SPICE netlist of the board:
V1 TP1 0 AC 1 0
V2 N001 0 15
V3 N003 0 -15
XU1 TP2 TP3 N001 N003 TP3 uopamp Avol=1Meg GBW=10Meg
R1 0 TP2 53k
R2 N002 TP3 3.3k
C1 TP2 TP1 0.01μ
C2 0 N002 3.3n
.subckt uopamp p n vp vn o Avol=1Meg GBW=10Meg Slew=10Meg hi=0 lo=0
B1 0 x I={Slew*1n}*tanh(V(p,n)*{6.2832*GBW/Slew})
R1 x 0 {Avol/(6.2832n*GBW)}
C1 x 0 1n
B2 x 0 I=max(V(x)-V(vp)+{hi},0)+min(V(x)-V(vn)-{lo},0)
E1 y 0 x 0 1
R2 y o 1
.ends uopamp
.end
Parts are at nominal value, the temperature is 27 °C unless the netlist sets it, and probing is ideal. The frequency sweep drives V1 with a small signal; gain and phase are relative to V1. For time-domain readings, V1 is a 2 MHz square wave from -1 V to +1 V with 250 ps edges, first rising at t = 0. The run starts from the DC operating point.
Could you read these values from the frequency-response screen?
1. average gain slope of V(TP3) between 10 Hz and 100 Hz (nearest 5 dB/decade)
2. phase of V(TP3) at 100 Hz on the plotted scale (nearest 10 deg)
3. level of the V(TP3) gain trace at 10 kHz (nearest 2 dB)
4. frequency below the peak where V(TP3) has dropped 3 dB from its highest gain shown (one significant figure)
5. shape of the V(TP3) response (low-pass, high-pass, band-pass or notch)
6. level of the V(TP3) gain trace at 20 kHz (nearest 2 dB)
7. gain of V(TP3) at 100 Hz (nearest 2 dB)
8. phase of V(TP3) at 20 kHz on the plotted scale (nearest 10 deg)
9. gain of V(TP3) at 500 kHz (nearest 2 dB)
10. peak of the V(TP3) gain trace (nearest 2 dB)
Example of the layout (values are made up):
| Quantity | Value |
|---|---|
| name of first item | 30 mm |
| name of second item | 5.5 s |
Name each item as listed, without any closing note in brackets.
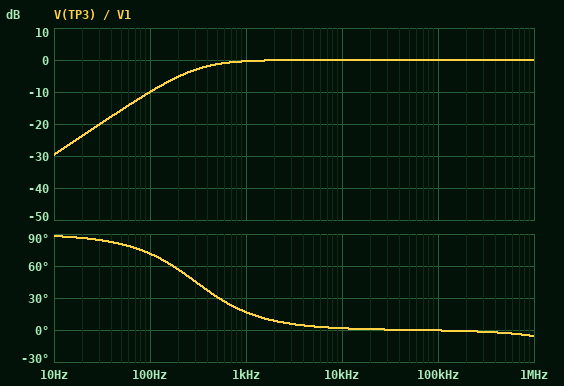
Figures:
| Quantity | Value |
|---|---|
| average gain slope of V(TP3) between 10 Hz and 100 Hz | 20 dB/decade |
| phase of V(TP3) at 100 Hz on the plotted scale | 70 deg |
| level of the V(TP3) gain trace at 10 kHz | 0 dB |
| frequency below the peak where V(TP3) has dropped 3 dB from its highest gain shown | 300 Hz |
| shape of the V(TP3) response | high-pass |
| level of the V(TP3) gain trace at 20 kHz | 0 dB |
| gain of V(TP3) at 100 Hz | -10 dB |
| phase of V(TP3) at 20 kHz on the plotted scale | 0 deg |
| gain of V(TP3) at 500 kHz | 0 dB |
| peak of the V(TP3) gain trace | 0 dB |
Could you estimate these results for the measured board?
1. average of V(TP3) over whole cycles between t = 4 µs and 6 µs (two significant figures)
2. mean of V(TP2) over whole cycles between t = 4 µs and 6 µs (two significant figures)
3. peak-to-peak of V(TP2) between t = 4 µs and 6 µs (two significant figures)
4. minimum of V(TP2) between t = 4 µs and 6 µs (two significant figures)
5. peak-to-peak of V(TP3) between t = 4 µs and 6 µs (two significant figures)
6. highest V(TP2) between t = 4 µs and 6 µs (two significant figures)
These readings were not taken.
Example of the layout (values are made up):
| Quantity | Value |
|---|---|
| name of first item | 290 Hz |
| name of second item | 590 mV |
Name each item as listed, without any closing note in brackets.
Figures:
| Quantity | Value |
|---|---|
| average of V(TP3) over whole cycles between t = 4 µs and 6 µs | 990 mV |
| mean of V(TP2) over whole cycles between t = 4 µs and 6 µs | 990 mV |
| peak-to-peak of V(TP2) between t = 4 µs and 6 µs | 2.0 V |
| minimum of V(TP2) between t = 4 µs and 6 µs | -11 mV |
| peak-to-peak of V(TP3) between t = 4 µs and 6 µs | 2.0 V |
| highest V(TP2) between t = 4 µs and 6 µs | 2.0 V |
